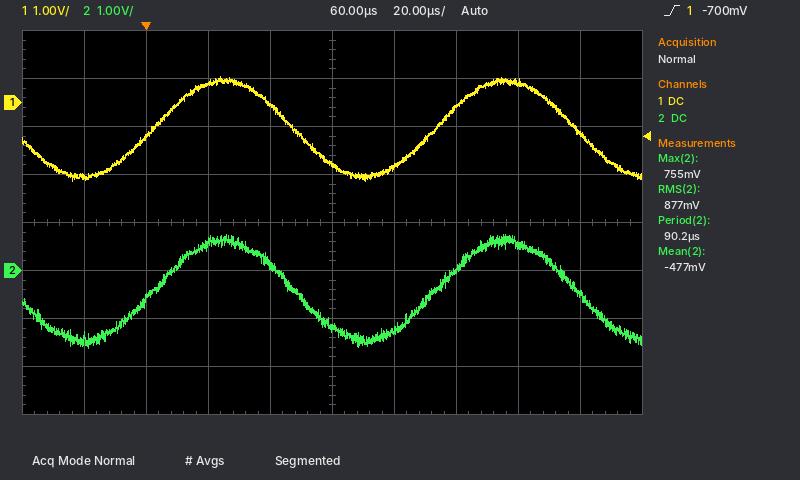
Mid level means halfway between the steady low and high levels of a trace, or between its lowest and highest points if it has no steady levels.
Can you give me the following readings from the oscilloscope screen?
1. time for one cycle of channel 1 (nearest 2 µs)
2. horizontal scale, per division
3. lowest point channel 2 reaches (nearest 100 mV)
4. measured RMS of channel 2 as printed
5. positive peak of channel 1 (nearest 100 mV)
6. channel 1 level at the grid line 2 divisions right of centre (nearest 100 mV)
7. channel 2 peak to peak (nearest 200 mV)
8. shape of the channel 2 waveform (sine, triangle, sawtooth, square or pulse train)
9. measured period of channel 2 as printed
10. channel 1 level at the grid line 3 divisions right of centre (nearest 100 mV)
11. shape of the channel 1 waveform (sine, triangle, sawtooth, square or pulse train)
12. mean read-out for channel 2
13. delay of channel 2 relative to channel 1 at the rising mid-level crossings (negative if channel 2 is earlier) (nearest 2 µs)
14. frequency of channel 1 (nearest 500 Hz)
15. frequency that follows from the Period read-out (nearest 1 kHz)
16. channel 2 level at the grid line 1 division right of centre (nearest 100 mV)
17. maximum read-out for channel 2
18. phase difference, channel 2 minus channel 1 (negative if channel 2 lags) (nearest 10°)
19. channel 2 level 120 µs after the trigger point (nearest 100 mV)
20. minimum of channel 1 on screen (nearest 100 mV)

92 µs
20 µs
-1.6 V
877 mV
500 mV
-100 mV
2.4 V
sine
90.2 µs
400 mV
sine
-477 mV
0 µs
11.0 kHz
11 kHz
-1.2 V
755 mV
0°
500 mV
-1.6 V
